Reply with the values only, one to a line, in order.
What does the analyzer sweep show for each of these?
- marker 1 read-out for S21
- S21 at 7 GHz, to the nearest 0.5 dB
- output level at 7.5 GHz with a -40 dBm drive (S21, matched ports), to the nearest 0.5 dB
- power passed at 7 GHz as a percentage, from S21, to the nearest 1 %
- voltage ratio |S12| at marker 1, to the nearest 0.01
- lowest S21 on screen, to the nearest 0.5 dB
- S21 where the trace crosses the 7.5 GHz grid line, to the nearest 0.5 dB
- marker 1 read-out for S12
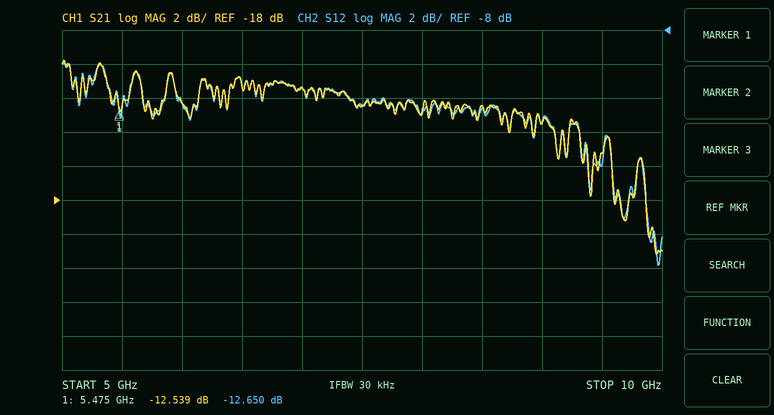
-12.539 dB
-11.5 dB
-52.5 dBm
7 %
0.23
-21.0 dB
-12.5 dB
-12.650 dB
